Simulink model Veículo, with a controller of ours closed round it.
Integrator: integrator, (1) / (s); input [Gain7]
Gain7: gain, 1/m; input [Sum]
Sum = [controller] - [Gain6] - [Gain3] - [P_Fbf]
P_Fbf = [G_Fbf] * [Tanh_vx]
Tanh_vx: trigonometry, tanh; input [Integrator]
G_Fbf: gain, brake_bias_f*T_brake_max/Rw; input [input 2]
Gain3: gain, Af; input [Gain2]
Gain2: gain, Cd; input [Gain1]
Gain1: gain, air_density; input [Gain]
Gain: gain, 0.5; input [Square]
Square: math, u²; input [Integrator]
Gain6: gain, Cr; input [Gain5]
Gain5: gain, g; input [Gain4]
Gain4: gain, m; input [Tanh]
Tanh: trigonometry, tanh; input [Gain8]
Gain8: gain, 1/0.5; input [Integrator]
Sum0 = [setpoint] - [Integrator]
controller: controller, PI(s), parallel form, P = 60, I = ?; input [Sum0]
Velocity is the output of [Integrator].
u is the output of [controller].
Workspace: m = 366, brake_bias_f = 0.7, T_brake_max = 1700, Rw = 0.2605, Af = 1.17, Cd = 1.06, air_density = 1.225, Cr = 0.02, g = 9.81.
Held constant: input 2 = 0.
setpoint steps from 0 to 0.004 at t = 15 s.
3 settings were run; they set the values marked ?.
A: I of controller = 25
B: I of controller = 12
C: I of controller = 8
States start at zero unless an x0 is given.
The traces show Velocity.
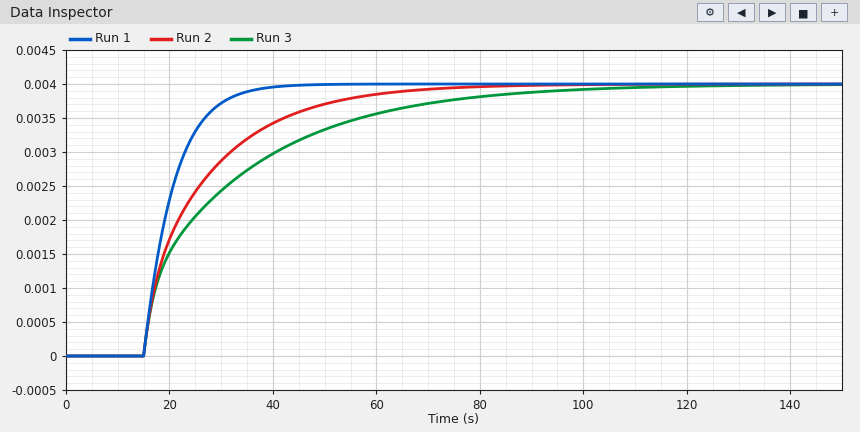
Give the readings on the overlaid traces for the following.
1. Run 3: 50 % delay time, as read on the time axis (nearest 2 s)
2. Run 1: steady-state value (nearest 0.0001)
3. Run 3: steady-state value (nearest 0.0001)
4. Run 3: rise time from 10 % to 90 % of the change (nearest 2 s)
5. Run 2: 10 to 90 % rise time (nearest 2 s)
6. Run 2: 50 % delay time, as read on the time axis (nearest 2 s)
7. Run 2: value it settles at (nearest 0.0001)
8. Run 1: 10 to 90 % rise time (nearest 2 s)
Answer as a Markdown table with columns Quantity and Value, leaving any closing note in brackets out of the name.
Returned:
| Quantity | Value |
|---|---|
| Run 3: 50 % delay time, as read on the time axis | 24 s |
| Run 1: steady-state value | 0.0040 |
| Run 3: steady-state value | 0.0040 |
| Run 3: rise time from 10 % to 90 % of the change | 46 s |
| Run 2: 10 to 90 % rise time | 30 s |
| Run 2: 50 % delay time, as read on the time axis | 22 s |
| Run 2: value it settles at | 0.0040 |
| Run 1: 10 to 90 % rise time | 12 s |
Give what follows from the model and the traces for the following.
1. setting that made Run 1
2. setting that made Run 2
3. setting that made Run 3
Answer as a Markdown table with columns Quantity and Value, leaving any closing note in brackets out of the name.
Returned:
| Quantity | Value |
|---|---|
| setting that made Run 1 | A |
| setting that made Run 2 | B |
| setting that made Run 3 | C |
